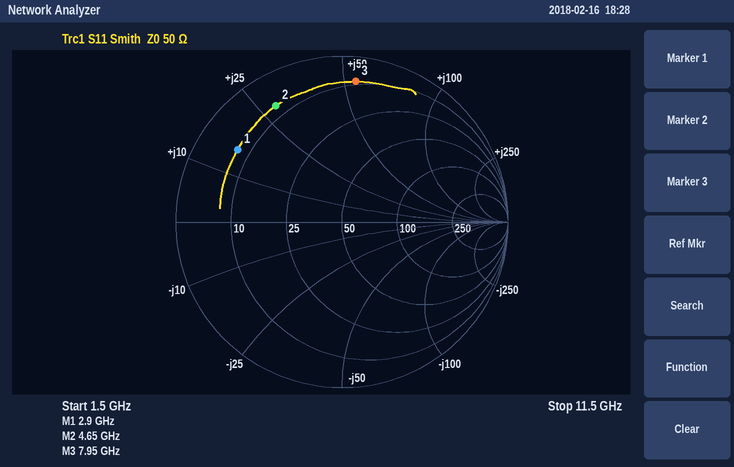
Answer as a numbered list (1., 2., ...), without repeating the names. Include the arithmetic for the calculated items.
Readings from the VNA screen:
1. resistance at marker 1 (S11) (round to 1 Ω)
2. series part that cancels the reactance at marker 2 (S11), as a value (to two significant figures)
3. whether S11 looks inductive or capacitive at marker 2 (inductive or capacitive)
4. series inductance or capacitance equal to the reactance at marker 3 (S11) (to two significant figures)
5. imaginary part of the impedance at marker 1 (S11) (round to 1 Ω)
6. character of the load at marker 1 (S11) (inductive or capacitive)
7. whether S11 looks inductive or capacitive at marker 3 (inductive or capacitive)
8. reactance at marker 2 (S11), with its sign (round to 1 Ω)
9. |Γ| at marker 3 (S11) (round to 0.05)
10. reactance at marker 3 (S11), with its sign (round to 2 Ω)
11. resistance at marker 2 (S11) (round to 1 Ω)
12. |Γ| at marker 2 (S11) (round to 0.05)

1. 7 Ω
2. C = 1/(2π × 4.65 GHz × 29 Ω) ≈ 1.2 pF
3. inductive
4. L = 54 Ω/(2π × 7.95 GHz) ≈ 1.1 nH
5. +15 Ω
6. inductive
7. inductive
8. +29 Ω
9. 0.85
10. +54 Ω
11. 7 Ω
12. 0.80
